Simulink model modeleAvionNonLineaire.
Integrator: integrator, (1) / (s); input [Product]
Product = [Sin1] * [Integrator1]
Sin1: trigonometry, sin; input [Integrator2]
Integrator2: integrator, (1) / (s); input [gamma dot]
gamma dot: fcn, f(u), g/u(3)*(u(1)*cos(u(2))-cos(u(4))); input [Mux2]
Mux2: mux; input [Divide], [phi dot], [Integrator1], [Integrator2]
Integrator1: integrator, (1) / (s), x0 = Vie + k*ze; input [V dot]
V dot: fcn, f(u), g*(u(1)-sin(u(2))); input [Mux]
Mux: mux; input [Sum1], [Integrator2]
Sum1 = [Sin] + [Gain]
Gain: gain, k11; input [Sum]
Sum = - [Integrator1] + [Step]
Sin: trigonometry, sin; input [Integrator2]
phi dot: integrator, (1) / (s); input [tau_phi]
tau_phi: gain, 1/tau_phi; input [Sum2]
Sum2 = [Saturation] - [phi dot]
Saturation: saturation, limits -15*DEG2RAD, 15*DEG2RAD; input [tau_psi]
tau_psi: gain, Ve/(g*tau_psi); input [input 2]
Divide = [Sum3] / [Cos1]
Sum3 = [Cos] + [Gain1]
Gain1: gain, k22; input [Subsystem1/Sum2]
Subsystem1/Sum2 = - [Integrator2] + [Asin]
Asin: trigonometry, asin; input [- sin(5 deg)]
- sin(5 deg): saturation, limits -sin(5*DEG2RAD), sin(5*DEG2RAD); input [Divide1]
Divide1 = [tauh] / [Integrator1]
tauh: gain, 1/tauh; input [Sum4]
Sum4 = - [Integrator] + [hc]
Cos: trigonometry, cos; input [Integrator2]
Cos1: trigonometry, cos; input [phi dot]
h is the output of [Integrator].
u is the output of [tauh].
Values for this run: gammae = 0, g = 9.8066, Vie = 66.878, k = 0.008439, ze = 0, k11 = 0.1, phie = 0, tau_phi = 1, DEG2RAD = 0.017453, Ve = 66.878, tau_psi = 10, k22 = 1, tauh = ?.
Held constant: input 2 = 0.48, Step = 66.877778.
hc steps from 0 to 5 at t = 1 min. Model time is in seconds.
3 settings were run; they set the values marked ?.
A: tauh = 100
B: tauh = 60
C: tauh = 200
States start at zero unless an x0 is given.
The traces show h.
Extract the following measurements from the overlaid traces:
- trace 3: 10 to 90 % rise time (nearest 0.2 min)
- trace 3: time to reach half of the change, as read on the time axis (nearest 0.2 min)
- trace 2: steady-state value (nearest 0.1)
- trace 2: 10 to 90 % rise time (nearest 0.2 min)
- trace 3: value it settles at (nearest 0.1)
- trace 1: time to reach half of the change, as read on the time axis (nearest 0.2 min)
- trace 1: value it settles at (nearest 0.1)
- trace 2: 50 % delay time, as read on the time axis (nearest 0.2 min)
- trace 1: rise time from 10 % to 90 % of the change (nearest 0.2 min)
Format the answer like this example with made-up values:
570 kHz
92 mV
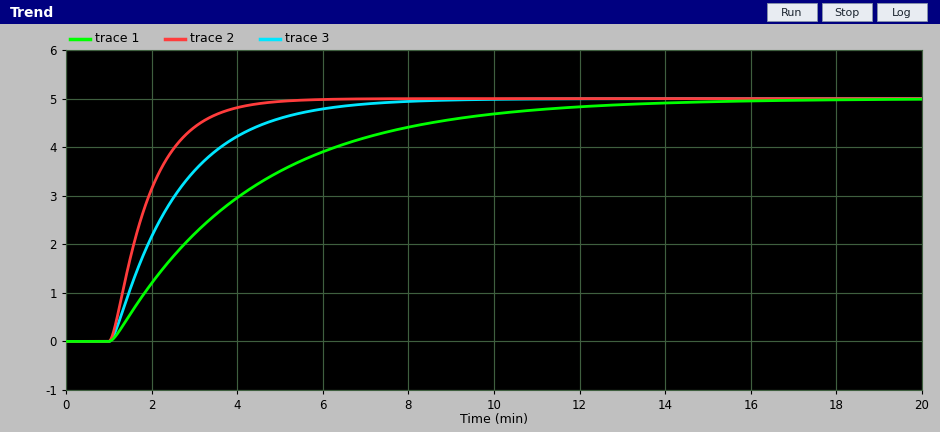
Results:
3.4 min
2.2 min
5.0
2.0 min
5.0
3.4 min
5.0
1.8 min
7.0 min
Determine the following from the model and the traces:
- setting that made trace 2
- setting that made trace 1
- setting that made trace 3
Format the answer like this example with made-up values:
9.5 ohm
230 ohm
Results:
B
C
A
